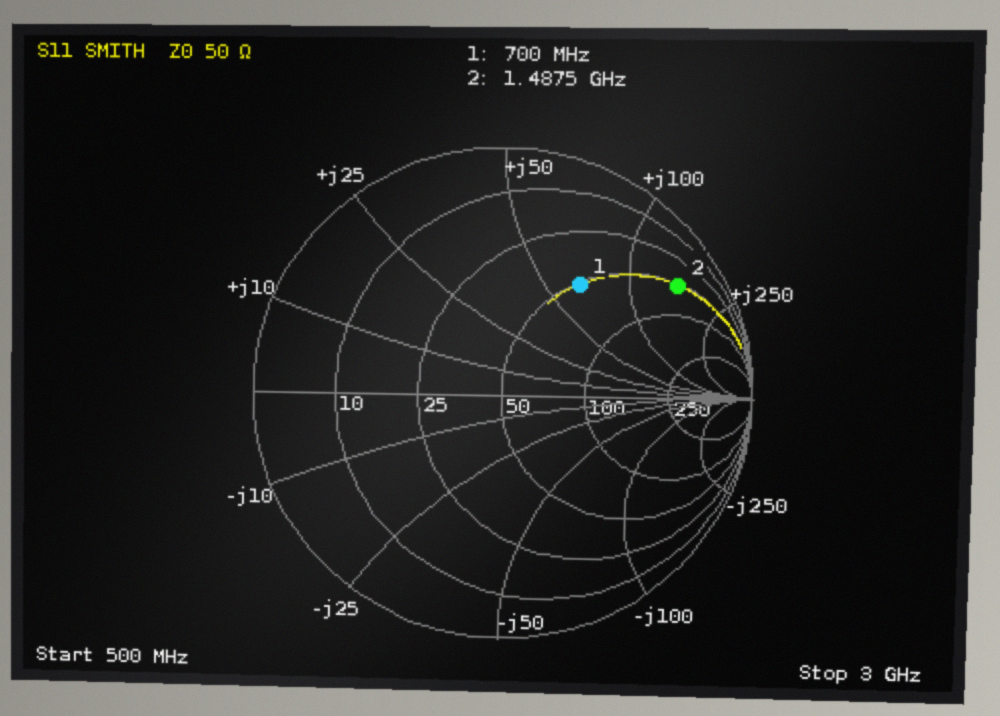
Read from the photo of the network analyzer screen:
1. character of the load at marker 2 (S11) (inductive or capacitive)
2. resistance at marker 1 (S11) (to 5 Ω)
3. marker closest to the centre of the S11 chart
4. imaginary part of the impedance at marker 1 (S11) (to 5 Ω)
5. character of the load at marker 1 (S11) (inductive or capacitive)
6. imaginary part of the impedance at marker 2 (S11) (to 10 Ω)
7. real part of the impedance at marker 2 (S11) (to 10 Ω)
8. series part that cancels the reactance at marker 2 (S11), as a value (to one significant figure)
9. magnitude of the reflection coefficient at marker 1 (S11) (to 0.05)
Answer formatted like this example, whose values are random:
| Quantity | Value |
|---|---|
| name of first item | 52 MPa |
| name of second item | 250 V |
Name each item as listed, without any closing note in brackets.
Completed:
| Quantity | Value |
|---|---|
| character of the load at marker 2 (S11) | inductive |
| resistance at marker 1 (S11) | 50 Ω |
| marker closest to the centre of the S11 chart | marker 1 |
| imaginary part of the impedance at marker 1 (S11) | +65 Ω |
| character of the load at marker 1 (S11) | inductive |
| imaginary part of the impedance at marker 2 (S11) | +150 Ω |
| real part of the impedance at marker 2 (S11) | 50 Ω |
| series part that cancels the reactance at marker 2 (S11), as a value | 700 fF |
| magnitude of the reflection coefficient at marker 1 (S11) | 0.55 |
